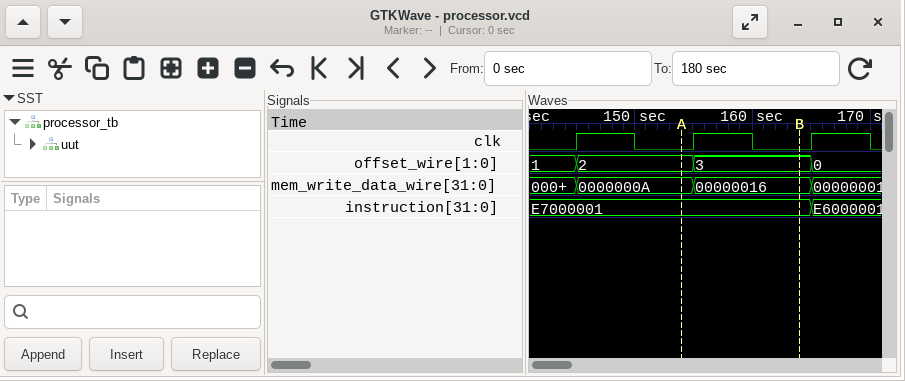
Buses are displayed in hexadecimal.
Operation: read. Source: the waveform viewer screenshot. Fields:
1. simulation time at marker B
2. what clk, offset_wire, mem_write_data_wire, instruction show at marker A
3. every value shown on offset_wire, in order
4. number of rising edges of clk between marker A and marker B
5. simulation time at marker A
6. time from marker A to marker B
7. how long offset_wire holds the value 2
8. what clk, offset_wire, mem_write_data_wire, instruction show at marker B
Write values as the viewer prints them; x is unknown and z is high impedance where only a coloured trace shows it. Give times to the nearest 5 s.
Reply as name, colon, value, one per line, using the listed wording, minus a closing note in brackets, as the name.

simulation time at marker B: 165 s
what clk, offset_wire, mem_write_data_wire, instruction show at marker A: clk=0, offset_wire=2, mem_write_data_wire=0000000A, instruction=E7000001
every value shown on offset_wire, in order: 1, 2, 3, 0
number of rising edges of clk between marker A and marker B: 1
simulation time at marker A: 155 s
time from marker A to marker B: 10 s
how long offset_wire holds the value 2: 10 s
what clk, offset_wire, mem_write_data_wire, instruction show at marker B: clk=0, offset_wire=3, mem_write_data_wire=00000016, instruction=E7000001
